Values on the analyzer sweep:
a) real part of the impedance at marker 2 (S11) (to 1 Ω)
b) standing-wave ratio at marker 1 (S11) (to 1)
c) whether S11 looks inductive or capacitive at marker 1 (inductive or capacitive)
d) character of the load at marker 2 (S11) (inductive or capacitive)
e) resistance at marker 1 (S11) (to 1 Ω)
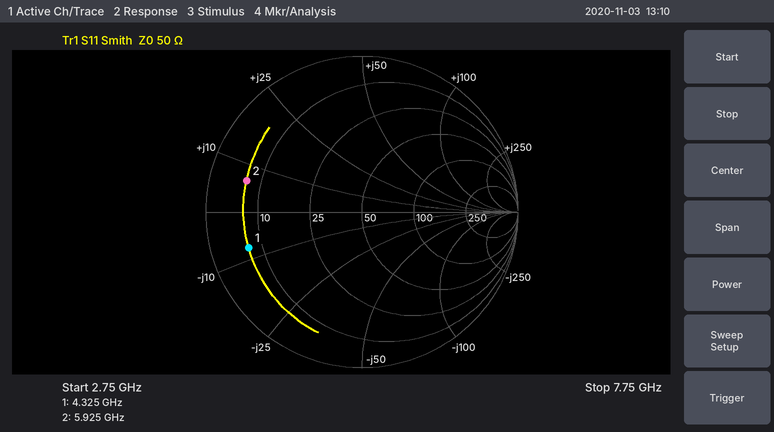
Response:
7 Ω
7
capacitive
inductive
7 Ω
